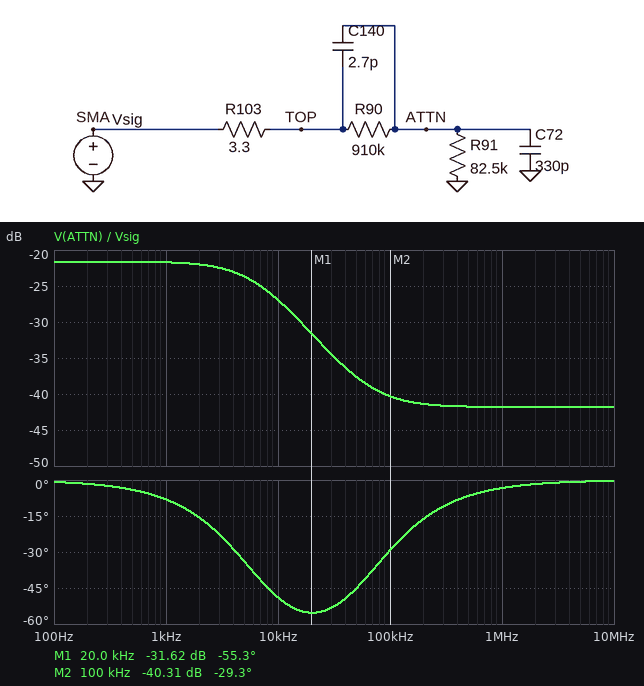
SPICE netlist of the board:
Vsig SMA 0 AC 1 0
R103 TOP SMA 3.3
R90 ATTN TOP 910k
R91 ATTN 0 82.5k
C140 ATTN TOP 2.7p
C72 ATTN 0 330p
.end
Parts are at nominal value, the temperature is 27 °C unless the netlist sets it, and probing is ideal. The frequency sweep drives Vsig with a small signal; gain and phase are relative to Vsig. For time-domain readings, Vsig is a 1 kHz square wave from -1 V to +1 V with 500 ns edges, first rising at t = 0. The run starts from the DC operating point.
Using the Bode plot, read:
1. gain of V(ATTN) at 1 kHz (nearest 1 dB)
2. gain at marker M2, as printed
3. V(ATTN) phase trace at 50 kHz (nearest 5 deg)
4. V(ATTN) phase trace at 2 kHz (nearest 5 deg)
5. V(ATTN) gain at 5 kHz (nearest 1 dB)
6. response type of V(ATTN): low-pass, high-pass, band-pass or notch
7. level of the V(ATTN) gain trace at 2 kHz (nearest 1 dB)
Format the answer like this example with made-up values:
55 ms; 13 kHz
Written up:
-22 dB; -40.31 dB; -45 deg; -15 deg; -24 dB; low-pass; -22 dB
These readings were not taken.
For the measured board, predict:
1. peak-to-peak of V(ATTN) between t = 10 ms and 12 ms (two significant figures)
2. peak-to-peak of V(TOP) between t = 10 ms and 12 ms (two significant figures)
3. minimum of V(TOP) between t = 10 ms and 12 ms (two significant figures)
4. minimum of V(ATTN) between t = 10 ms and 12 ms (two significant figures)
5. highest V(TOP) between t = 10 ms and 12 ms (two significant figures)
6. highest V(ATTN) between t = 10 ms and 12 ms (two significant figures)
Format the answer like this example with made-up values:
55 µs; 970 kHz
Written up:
170 mV; 2.0 V; -1.0 V; -83 mV; 1.0 V; 83 mV
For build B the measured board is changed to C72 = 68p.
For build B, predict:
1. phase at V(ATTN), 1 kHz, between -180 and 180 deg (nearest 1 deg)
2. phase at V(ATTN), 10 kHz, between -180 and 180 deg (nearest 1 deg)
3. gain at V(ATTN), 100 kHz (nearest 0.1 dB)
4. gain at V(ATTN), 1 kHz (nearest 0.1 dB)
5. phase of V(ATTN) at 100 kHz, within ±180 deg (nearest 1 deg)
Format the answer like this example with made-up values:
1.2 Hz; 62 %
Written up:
-1 deg; -10 deg; -27.2 dB; -21.6 dB; -16 deg
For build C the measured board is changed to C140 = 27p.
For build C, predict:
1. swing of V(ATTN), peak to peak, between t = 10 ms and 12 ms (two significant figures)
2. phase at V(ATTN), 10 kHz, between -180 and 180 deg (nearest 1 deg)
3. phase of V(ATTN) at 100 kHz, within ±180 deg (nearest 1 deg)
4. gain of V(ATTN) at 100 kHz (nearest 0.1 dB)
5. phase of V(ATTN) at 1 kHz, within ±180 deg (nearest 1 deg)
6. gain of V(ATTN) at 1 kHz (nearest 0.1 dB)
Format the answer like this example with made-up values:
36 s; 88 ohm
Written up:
170 mV; -2 deg; 0 deg; -22.4 dB; -1 deg; -21.6 dB
